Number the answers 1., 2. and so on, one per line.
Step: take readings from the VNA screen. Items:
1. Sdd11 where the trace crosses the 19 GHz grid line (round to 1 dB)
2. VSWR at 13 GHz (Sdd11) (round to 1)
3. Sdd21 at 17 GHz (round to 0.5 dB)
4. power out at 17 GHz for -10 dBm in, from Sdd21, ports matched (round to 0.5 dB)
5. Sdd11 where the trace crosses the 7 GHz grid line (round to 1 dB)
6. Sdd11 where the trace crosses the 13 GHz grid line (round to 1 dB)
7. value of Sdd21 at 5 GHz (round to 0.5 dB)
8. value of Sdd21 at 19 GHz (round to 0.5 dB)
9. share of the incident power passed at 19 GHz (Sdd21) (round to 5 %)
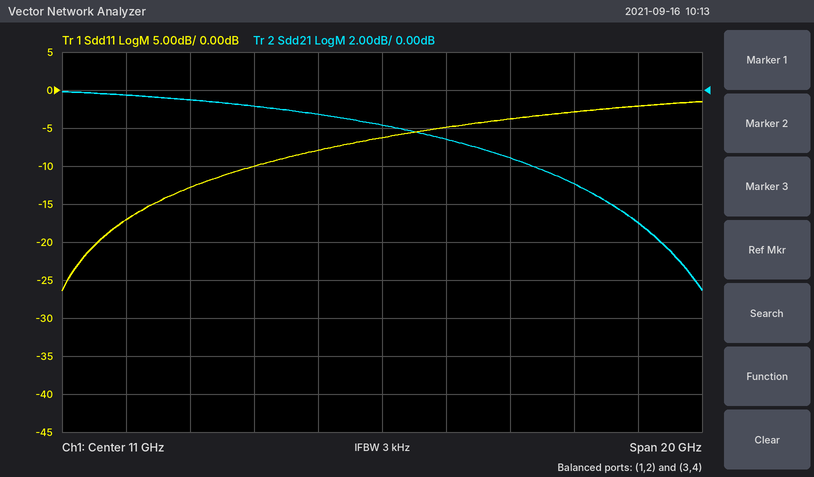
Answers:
1. -2 dB
2. 4
3. -5.0 dB
4. -15.0 dBm
5. -10 dB
6. -5 dB
7. -0.5 dB
8. -7.0 dB
9. 20 %
